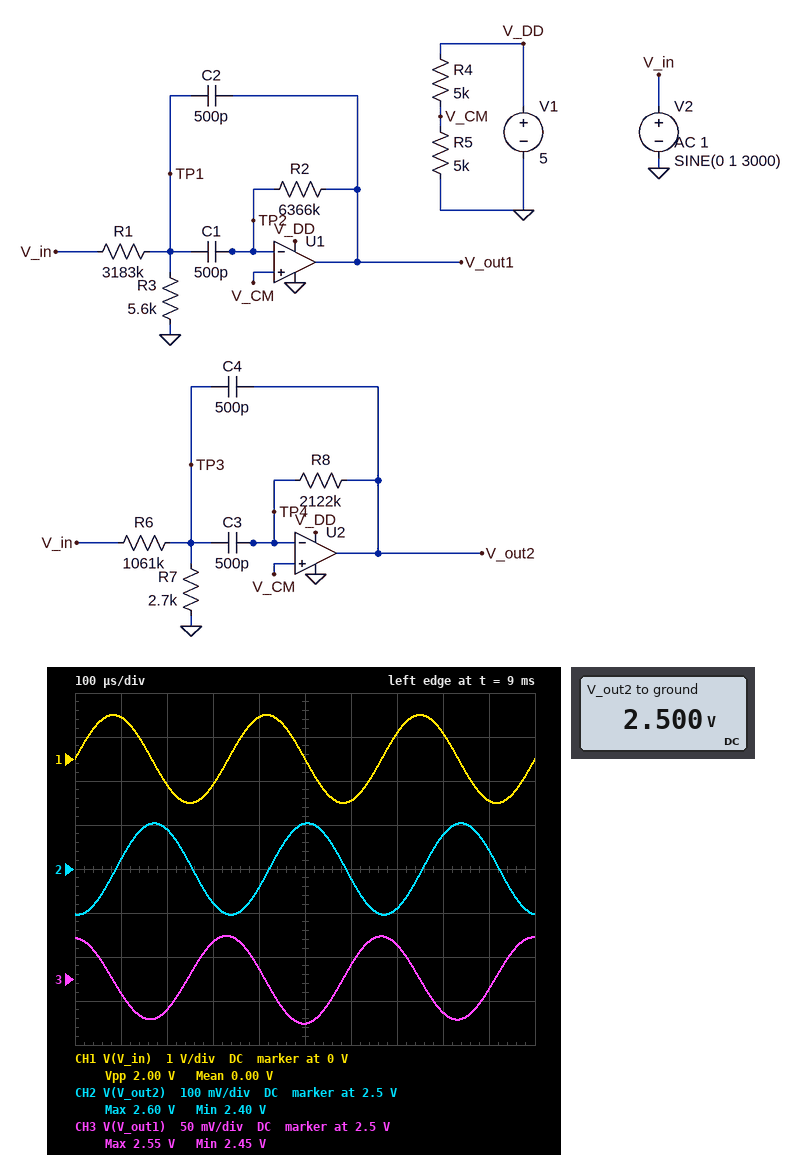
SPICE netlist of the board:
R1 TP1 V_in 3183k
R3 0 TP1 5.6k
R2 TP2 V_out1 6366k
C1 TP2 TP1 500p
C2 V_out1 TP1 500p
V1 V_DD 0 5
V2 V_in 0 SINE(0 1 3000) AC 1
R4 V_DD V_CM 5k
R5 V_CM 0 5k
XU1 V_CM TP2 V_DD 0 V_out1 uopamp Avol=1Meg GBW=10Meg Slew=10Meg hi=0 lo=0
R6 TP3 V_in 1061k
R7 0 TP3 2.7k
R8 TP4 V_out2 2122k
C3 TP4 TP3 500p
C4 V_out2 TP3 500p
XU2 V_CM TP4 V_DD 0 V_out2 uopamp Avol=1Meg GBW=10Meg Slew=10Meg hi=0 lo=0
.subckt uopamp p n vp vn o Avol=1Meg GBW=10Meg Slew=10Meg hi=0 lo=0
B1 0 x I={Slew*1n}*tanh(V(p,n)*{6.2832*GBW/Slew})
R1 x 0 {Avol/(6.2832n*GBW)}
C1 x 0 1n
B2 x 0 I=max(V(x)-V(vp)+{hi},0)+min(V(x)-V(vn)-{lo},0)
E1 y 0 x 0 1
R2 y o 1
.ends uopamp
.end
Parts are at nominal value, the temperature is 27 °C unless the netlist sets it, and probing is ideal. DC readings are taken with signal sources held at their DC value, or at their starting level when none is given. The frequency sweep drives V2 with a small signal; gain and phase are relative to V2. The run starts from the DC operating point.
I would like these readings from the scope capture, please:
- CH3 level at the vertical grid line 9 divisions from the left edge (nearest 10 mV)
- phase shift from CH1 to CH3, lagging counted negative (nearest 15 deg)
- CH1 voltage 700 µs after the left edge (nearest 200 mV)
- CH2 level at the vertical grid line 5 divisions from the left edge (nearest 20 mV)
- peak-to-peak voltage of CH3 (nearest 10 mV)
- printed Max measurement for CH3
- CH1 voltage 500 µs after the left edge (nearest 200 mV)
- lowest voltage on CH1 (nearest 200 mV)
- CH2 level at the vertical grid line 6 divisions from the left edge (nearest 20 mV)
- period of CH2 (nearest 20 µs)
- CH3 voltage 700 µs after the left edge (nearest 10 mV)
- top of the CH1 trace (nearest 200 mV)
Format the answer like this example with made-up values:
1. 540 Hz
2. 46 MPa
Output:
1. 2.49 V
2. 90 deg
3. 600 mV
4. 2.60 V
5. 100 mV
6. 2.55 V
7. 0 V
8. -1.0 V
9. 2.48 V
10. 340 µs
11. 2.54 V
12. 1.0 V
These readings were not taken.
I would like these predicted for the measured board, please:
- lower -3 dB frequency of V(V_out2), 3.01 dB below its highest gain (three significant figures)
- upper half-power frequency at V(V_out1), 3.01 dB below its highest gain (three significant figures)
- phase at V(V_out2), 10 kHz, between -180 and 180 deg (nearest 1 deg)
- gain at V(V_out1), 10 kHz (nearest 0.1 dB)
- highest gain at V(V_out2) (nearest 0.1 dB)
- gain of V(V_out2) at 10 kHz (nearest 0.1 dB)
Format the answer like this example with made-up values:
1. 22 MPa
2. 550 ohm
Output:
1. 4.04 kHz
2. 1.73 kHz
3. 92 deg
4. -39.8 dB
5. 0 dB
6. -28.9 dB
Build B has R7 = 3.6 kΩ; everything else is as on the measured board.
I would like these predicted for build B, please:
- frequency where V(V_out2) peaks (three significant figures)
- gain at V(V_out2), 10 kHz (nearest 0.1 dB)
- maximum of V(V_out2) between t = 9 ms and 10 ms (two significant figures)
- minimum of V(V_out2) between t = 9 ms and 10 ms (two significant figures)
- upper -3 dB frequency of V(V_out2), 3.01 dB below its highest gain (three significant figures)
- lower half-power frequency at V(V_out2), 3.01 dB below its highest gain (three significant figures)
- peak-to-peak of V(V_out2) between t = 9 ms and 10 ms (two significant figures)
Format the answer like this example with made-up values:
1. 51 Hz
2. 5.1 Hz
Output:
1. 3.63 kHz
2. -29.3 dB
3. 2.7 V
4. 2.3 V
5. 3.78 kHz
6. 3.49 kHz
7. 420 mV
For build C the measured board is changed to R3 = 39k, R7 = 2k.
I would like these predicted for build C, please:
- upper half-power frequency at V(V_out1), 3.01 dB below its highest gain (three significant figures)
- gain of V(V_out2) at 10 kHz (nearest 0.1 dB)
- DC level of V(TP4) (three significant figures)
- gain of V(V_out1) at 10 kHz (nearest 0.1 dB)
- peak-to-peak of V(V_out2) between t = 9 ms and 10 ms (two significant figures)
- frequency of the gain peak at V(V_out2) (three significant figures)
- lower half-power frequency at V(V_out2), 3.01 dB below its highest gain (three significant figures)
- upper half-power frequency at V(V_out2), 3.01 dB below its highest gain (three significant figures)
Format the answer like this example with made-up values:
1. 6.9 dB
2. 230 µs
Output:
1. 694 Hz
2. -28.3 dB
3. 2.50 V
4. -40.0 dB
5. 120 mV
6. 4.85 kHz
7. 4.71 kHz
8. 5.00 kHz
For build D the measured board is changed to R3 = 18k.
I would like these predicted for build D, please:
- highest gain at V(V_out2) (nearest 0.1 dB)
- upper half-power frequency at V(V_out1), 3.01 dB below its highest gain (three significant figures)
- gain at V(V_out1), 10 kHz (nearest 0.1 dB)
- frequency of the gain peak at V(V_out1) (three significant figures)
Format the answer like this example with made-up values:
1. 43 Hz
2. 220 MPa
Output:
1. 0 dB
2. 993 Hz
3. -39.9 dB
4. 942 Hz
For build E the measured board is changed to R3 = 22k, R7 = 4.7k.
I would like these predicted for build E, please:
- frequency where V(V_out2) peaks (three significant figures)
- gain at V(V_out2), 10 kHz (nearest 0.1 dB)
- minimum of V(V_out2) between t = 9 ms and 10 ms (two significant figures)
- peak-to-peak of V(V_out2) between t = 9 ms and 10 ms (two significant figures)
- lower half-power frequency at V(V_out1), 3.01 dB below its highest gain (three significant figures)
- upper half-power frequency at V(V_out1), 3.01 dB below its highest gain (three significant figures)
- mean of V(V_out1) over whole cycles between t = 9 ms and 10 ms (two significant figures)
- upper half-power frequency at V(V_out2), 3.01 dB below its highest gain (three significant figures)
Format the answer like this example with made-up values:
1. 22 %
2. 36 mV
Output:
1. 3.18 kHz
2. -29.6 dB
3. 1.9 V
4. 1.2 V
5. 804 Hz
6. 904 Hz
7. 2.5 V
8. 3.34 kHz
